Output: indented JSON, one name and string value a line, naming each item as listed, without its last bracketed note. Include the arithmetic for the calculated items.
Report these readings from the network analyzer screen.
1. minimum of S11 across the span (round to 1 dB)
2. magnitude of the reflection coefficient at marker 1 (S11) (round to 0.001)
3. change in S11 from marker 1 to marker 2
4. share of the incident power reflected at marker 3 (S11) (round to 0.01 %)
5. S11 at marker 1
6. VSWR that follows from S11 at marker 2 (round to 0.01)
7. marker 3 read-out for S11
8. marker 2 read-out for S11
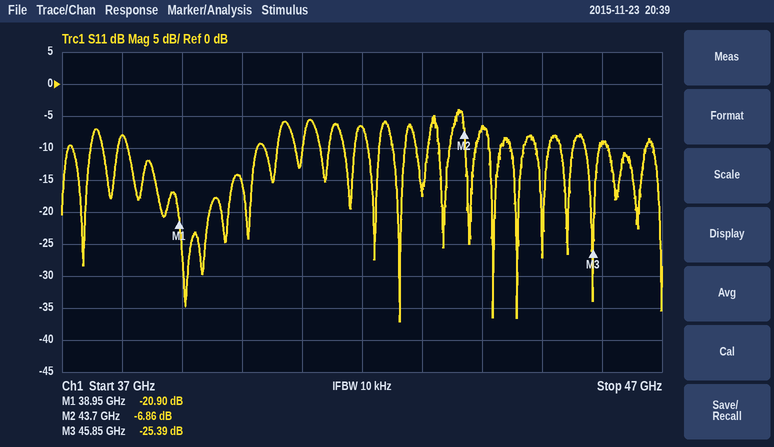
{
  "minimum of S11 across the span": "-37 dB",
  "magnitude of the reflection coefficient at marker 1 (S11)": "10^(-20.9/20) ≈ 0.090",
  "change in S11 from marker 1 to marker 2": "-6.86 − (-20.9) = 14.04 dB",
  "share of the incident power reflected at marker 3 (S11)": "10^(-25.39/10) ≈ 0.29 %",
  "S11 at marker 1": "-20.90 dB",
  "VSWR that follows from S11 at marker 2": "(1 + 0.4539)/(1 − 0.4539) ≈ 2.66",
  "marker 3 read-out for S11": "-25.39 dB",
  "marker 2 read-out for S11": "-6.86 dB"
}
